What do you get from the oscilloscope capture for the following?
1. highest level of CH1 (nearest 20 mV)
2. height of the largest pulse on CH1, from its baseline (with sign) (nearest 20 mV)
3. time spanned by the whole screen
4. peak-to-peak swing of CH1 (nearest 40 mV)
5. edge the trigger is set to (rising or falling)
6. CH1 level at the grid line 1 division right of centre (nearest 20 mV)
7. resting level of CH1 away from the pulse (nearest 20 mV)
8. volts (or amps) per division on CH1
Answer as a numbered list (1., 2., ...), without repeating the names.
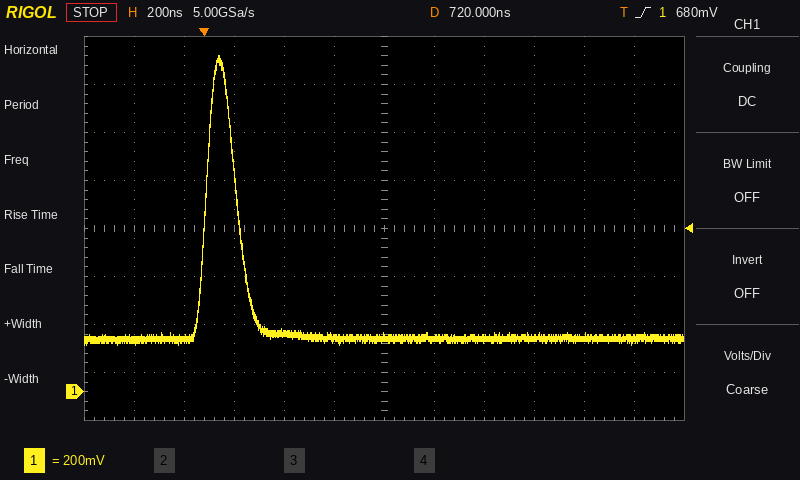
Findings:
1. 1.40 V
2. +1.18 V
3. 2.4 µs
4. 1.20 V
5. rising
6. 220 mV
7. 220 mV
8. 200 mV
